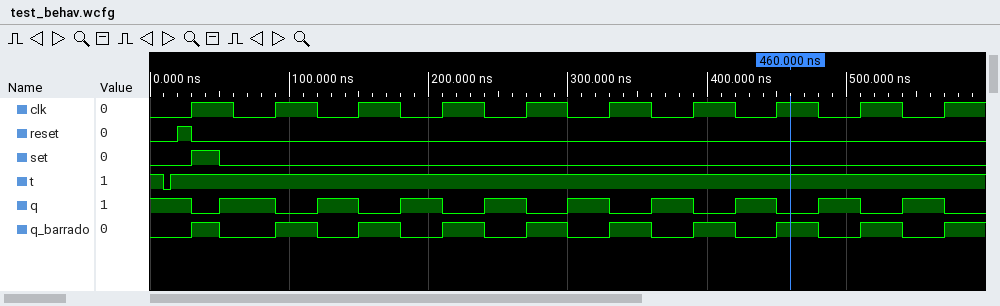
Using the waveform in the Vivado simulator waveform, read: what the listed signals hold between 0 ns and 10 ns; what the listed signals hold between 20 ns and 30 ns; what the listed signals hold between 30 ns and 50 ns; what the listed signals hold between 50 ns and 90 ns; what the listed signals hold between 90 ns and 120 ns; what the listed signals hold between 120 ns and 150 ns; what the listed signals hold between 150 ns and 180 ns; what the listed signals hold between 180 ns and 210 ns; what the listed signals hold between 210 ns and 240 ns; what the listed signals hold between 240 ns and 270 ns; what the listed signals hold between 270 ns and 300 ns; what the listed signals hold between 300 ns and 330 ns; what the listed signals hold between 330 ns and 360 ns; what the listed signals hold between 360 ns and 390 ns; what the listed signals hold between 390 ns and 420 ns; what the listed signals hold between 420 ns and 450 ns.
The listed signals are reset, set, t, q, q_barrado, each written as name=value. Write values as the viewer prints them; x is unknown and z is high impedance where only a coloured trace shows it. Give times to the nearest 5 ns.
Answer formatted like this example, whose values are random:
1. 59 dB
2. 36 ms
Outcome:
1. reset=0, set=0, t=1, q=1, q_barrado=0
2. reset=1, set=0, t=1, q=1, q_barrado=0
3. reset=0, set=1, t=1, q=0, q_barrado=1
4. reset=0, set=0, t=1, q=1, q_barrado=0
5. reset=0, set=0, t=1, q=0, q_barrado=1
6. reset=0, set=0, t=1, q=1, q_barrado=0
7. reset=0, set=0, t=1, q=0, q_barrado=1
8. reset=0, set=0, t=1, q=1, q_barrado=0
9. reset=0, set=0, t=1, q=0, q_barrado=1
10. reset=0, set=0, t=1, q=1, q_barrado=0
11. reset=0, set=0, t=1, q=0, q_barrado=1
12. reset=0, set=0, t=1, q=1, q_barrado=0
13. reset=0, set=0, t=1, q=0, q_barrado=1
14. reset=0, set=0, t=1, q=1, q_barrado=0
15. reset=0, set=0, t=1, q=0, q_barrado=1
16. reset=0, set=0, t=1, q=1, q_barrado=0
